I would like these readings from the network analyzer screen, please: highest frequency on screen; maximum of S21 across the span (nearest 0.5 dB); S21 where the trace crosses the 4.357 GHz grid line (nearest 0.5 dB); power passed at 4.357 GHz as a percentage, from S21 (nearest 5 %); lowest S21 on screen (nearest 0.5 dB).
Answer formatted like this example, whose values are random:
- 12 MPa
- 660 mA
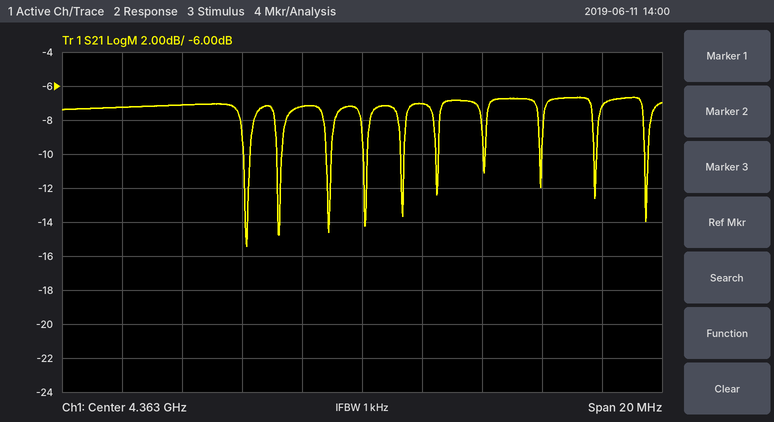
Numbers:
- 4.373 GHz
- -6.5 dB
- -7.0 dB
- 20 %
- -15.5 dB
